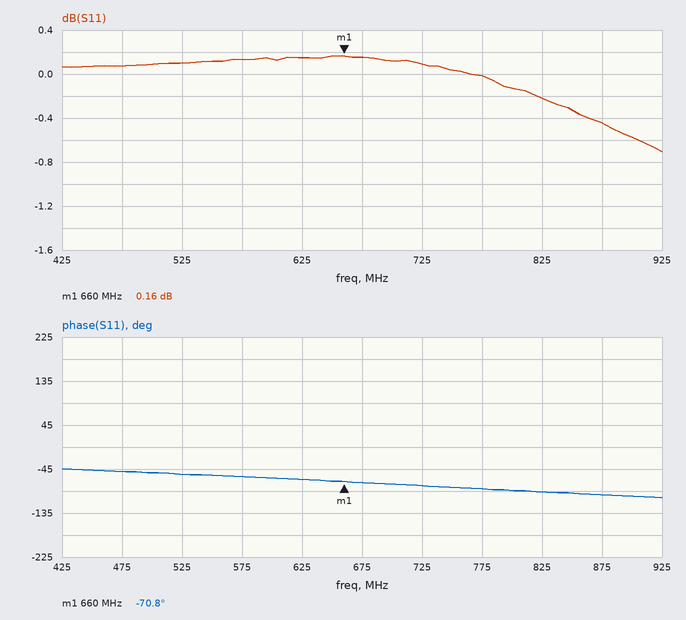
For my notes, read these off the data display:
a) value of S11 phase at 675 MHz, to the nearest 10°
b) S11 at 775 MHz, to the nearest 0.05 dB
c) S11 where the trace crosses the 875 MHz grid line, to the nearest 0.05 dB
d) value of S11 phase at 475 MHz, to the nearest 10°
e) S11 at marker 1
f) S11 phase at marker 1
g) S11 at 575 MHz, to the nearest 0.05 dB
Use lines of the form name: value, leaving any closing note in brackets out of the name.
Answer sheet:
value of S11 phase at 675 MHz, to the nearest 10°: -70°
S11 at 775 MHz, to the nearest 0.05 dB: 0.00 dB
S11 where the trace crosses the 875 MHz grid line, to the nearest 0.05 dB: -0.45 dB
value of S11 phase at 475 MHz, to the nearest 10°: -50°
S11 at marker 1: 0.16 dB
S11 phase at marker 1: -70.8°
S11 at 575 MHz, to the nearest 0.05 dB: 0.15 dB
